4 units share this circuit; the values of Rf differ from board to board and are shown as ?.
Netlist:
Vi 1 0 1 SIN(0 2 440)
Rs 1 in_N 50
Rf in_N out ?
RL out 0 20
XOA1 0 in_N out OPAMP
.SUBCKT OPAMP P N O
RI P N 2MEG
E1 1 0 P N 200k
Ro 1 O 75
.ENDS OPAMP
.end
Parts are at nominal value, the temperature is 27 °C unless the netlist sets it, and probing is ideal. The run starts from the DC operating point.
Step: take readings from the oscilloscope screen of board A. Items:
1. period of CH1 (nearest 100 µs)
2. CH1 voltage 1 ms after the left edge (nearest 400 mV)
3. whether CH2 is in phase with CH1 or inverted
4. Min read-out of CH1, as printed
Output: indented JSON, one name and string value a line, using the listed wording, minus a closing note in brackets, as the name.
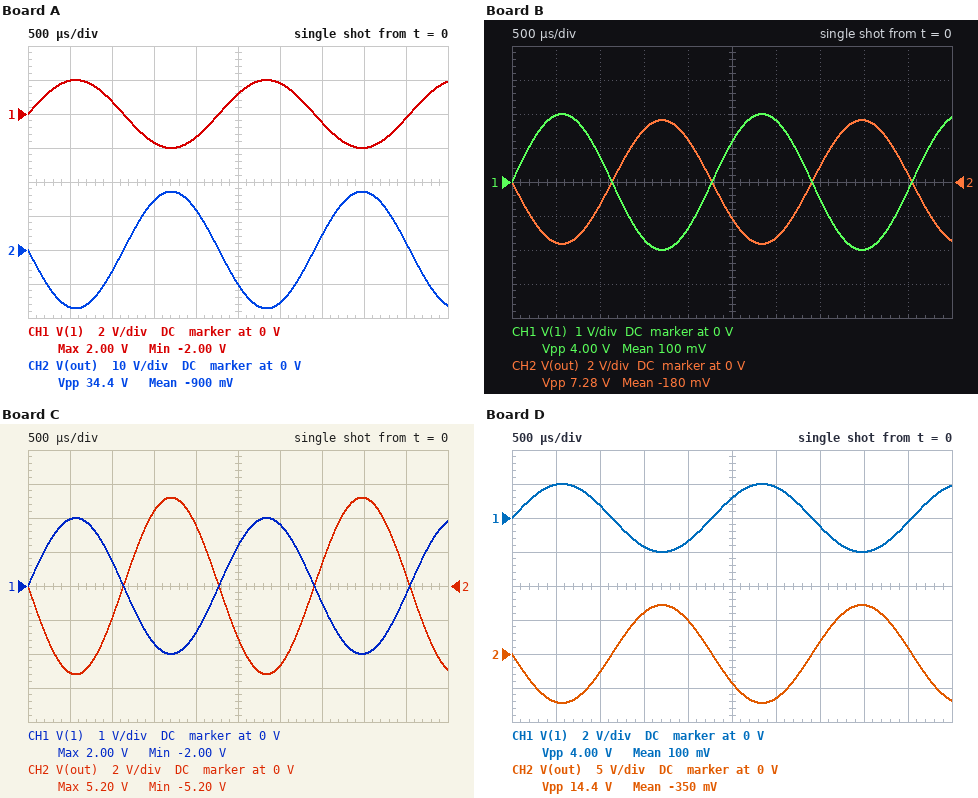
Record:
{
  "period of CH1": "2.3 ms",
  "CH1 voltage 1 ms after the left edge": "800 mV",
  "whether CH2 is in phase with CH1 or inverted": "inverted",
  "Min read-out of CH1, as printed": "-2.00 V"
}
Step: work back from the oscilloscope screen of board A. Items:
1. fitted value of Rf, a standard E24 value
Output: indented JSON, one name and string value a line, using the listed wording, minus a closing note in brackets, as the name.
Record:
{
  "fitted value of Rf, a standard E24 value": "430 Ω"
}
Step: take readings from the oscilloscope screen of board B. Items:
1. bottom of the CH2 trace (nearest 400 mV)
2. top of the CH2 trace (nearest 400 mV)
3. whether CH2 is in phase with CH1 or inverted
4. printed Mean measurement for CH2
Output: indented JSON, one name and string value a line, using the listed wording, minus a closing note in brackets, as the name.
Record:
{
  "bottom of the CH2 trace": "-3.6 V",
  "top of the CH2 trace": "3.6 V",
  "whether CH2 is in phase with CH1 or inverted": "inverted",
  "printed Mean measurement for CH2": "-180 mV"
}
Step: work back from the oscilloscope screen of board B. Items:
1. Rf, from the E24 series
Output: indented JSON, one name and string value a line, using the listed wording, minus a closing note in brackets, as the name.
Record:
{
  "Rf, from the E24 series": "91 Ω"
}
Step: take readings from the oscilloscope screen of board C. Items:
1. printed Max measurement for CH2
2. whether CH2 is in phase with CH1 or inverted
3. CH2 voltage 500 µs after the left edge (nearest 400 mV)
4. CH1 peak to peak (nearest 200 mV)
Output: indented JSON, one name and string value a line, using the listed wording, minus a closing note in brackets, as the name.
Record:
{
  "printed Max measurement for CH2": "5.20 V",
  "whether CH2 is in phase with CH1 or inverted": "inverted",
  "CH2 voltage 500 µs after the left edge": "-5.2 V",
  "CH1 peak to peak": "4.0 V"
}
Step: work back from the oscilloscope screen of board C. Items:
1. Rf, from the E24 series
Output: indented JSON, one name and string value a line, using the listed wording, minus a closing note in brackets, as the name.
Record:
{
  "Rf, from the E24 series": "130 Ω"
}
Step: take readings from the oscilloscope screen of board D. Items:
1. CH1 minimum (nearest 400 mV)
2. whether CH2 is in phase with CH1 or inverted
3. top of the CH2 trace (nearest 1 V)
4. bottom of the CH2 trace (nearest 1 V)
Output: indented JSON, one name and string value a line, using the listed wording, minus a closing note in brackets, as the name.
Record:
{
  "CH1 minimum": "-2.0 V",
  "whether CH2 is in phase with CH1 or inverted": "inverted",
  "top of the CH2 trace": "7 V",
  "bottom of the CH2 trace": "-7 V"
}
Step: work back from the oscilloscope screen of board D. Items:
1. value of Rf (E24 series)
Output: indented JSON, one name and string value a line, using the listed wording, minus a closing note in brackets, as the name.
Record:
{
  "value of Rf": "180 Ω"
}
